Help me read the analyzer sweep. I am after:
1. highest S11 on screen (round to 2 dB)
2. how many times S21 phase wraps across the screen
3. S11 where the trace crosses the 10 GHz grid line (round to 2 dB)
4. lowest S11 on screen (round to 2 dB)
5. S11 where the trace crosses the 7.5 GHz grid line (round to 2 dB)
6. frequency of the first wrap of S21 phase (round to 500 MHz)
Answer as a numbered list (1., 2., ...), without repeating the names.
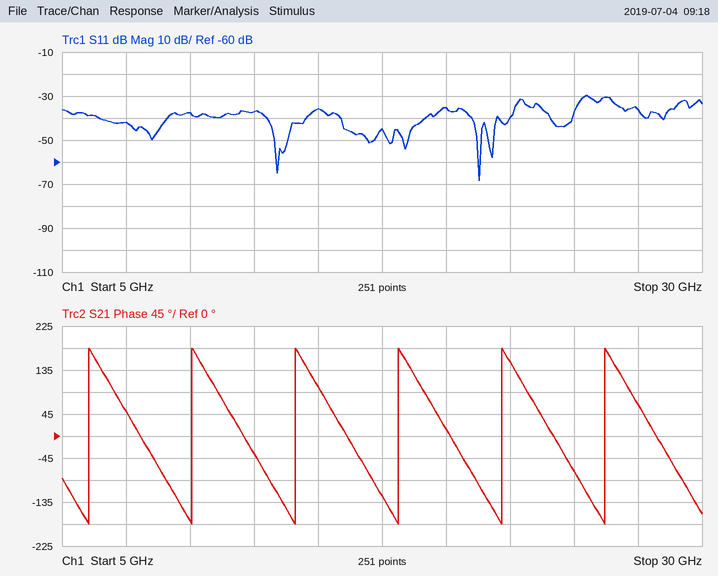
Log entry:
1. -30 dB
2. 6
3. -38 dB
4. -68 dB
5. -42 dB
6. 6.0 GHz
